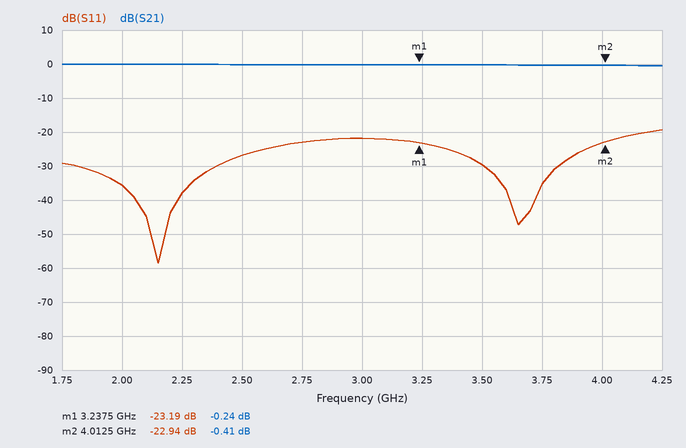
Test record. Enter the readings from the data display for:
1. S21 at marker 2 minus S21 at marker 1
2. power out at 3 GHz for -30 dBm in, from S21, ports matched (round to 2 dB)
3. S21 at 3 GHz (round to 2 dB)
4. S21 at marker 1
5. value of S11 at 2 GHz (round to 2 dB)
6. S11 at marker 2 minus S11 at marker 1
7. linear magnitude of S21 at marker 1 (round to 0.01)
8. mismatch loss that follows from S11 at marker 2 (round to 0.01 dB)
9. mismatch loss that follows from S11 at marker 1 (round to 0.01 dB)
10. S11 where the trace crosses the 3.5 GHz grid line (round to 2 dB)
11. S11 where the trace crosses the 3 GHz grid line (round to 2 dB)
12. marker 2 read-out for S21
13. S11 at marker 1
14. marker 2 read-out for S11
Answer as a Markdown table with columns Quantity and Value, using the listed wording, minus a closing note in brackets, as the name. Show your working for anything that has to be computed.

| Quantity | Value |
|---|---|
| S21 at marker 2 minus S21 at marker 1 | -0.41 − (-0.24) = -0.17 dB |
| power out at 3 GHz for -30 dBm in, from S21, ports matched | -30 dBm + (0 dB) = -30 dBm |
| S21 at 3 GHz | 0 dB |
| S21 at marker 1 | -0.24 dB |
| value of S11 at 2 GHz | -36 dB |
| S11 at marker 2 minus S11 at marker 1 | -22.94 − (-23.19) = 0.25 dB |
| linear magnitude of S21 at marker 1 | 10^(-0.24/20) ≈ 0.97 |
| mismatch loss that follows from S11 at marker 2 | −10 log10(1 − 10^(-22.94/10)) ≈ 0.02 dB |
| mismatch loss that follows from S11 at marker 1 | −10 log10(1 − 10^(-23.19/10)) ≈ 0.02 dB |
| S11 where the trace crosses the 3.5 GHz grid line | -30 dB |
| S11 where the trace crosses the 3 GHz grid line | -22 dB |
| marker 2 read-out for S21 | -0.41 dB |
| S11 at marker 1 | -23.19 dB |
| marker 2 read-out for S11 | -22.94 dB |
